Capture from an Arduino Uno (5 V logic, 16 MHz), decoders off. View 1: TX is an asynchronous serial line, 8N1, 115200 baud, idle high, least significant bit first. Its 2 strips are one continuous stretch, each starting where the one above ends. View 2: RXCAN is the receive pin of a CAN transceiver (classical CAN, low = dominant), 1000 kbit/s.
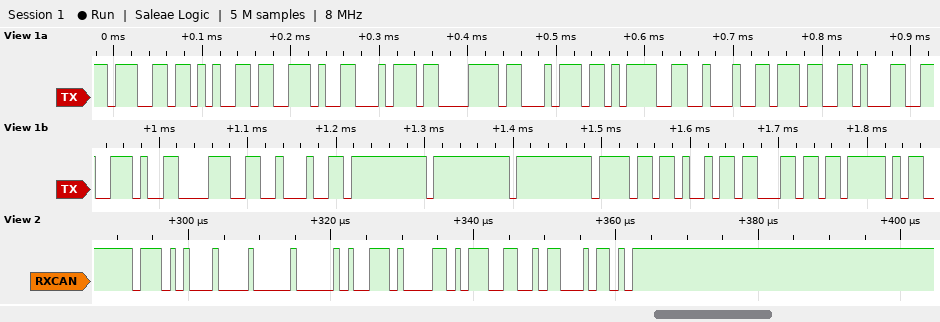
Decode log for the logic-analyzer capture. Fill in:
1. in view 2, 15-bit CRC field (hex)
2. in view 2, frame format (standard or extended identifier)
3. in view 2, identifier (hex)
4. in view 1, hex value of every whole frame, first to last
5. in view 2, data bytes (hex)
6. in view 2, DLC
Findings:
0x4B16
standard
0x751
67 65 2E 74 78 74 3D 22 37 31 2E 38 22 FF FF FF 6F 69 6C 5F
00 4E 86 B9
4
